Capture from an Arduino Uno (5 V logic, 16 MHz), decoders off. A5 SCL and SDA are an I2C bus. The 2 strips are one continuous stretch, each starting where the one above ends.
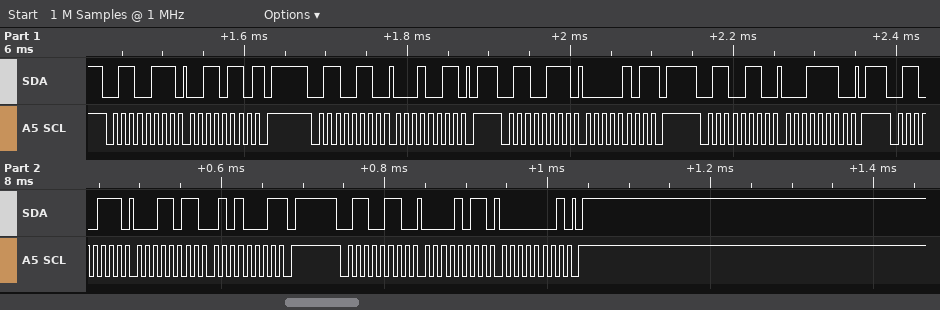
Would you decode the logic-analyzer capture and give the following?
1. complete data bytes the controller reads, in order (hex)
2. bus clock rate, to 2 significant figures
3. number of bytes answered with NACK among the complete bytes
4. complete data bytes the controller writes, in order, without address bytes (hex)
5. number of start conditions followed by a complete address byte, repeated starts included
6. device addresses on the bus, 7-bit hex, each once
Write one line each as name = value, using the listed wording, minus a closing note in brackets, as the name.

complete data bytes the controller reads, in order = 36 05 1B 51
bus clock rate, to 2 significant figures = 100 kHz
number of bytes answered with NACK among the complete bytes = 3
complete data bytes the controller writes, in order, without address bytes = 13 1E 0B 01
number of start conditions followed by a complete address byte, repeated starts included = 6
device addresses on the bus, 7-bit hex, each once = 0x33
